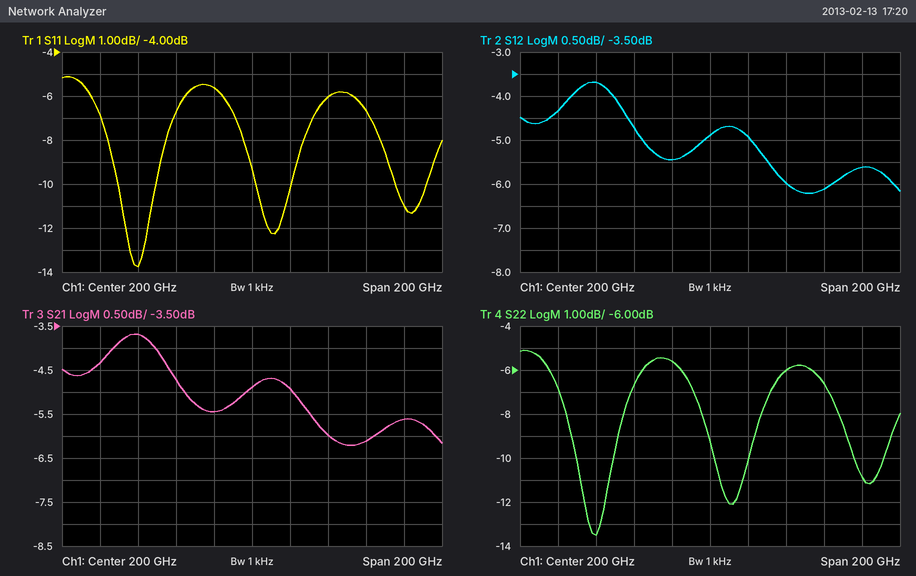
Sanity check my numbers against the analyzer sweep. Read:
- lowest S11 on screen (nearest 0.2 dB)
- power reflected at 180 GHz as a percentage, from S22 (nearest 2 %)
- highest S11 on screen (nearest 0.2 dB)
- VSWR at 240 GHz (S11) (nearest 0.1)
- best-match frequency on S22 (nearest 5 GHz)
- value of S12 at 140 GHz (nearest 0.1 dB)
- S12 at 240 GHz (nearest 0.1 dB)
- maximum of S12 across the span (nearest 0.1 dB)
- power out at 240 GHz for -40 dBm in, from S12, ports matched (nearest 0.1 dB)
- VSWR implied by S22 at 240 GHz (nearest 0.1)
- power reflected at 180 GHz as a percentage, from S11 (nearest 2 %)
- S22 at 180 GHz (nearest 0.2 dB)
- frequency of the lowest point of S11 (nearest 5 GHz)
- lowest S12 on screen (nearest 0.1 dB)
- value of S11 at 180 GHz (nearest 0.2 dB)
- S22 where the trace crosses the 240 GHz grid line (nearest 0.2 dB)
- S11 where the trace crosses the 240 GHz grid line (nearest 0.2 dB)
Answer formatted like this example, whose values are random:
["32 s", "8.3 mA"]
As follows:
["-13.8 dB", "28 %", "-5.2 dB", "3.0", "140 GHz", "-3.7 dB", "-6.0 dB", "-3.7 dB", "-46.0 dBm", "3.0", "28 %", "-5.6 dB", "140 GHz", "-6.2 dB", "-5.6 dB", "-6.0 dB", "-6.0 dB"]
